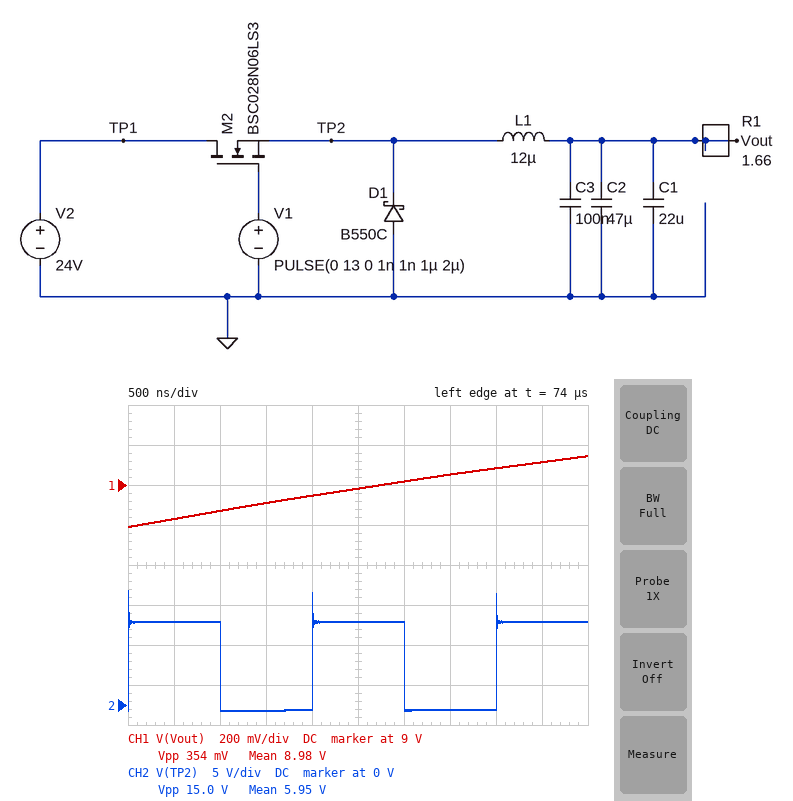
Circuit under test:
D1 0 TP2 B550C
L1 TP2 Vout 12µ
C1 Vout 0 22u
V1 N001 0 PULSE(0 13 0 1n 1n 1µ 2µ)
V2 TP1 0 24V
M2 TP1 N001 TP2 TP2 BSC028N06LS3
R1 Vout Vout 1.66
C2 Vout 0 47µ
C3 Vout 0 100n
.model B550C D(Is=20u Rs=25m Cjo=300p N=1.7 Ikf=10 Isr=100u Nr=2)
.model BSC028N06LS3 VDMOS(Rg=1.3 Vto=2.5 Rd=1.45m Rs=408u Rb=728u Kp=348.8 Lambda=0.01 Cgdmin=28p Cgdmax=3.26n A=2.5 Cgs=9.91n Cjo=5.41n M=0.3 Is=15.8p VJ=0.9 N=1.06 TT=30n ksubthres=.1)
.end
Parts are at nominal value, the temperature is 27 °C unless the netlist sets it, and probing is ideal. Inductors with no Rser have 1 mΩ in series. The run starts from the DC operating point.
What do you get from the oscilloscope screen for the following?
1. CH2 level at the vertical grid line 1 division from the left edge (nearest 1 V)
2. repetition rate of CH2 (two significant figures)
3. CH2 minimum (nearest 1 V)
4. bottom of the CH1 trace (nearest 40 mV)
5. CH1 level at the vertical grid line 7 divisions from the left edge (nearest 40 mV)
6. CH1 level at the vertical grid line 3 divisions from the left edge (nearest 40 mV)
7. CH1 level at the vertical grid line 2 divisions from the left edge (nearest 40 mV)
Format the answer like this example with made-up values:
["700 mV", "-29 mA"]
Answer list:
["10 V", "500 kHz", "-1 V", "8.80 V", "9.04 V", "8.92 V", "8.88 V"]
